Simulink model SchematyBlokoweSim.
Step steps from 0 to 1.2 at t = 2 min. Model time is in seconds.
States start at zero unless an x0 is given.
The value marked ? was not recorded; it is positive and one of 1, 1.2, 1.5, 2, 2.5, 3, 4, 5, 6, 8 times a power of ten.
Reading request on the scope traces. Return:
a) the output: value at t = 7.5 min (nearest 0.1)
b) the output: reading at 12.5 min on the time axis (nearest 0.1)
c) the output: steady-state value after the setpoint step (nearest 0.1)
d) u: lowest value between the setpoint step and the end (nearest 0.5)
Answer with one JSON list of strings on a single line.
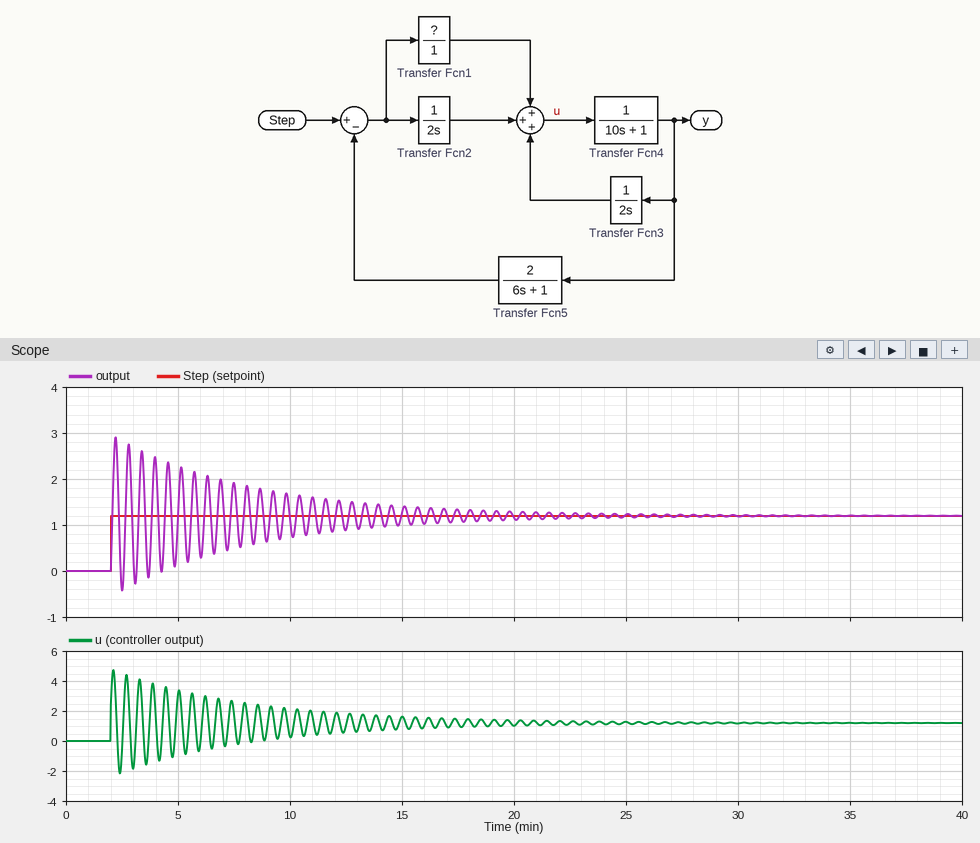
["1.9", "0.9", "1.2", "-2.0"]
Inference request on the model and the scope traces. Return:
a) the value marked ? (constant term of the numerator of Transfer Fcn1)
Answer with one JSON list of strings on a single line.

["2"]
